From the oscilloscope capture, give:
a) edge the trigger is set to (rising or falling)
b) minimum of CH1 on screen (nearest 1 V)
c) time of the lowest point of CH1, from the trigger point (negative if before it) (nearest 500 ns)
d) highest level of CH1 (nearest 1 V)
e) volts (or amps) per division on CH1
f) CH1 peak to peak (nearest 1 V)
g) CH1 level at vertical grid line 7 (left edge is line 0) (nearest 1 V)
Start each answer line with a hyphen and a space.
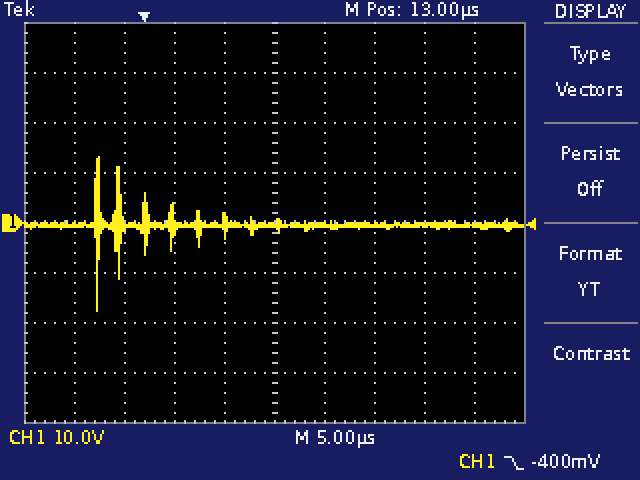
- falling
- -18 V
- -4.5 µs
- 13 V
- 10 V
- 31 V
- 0 V
